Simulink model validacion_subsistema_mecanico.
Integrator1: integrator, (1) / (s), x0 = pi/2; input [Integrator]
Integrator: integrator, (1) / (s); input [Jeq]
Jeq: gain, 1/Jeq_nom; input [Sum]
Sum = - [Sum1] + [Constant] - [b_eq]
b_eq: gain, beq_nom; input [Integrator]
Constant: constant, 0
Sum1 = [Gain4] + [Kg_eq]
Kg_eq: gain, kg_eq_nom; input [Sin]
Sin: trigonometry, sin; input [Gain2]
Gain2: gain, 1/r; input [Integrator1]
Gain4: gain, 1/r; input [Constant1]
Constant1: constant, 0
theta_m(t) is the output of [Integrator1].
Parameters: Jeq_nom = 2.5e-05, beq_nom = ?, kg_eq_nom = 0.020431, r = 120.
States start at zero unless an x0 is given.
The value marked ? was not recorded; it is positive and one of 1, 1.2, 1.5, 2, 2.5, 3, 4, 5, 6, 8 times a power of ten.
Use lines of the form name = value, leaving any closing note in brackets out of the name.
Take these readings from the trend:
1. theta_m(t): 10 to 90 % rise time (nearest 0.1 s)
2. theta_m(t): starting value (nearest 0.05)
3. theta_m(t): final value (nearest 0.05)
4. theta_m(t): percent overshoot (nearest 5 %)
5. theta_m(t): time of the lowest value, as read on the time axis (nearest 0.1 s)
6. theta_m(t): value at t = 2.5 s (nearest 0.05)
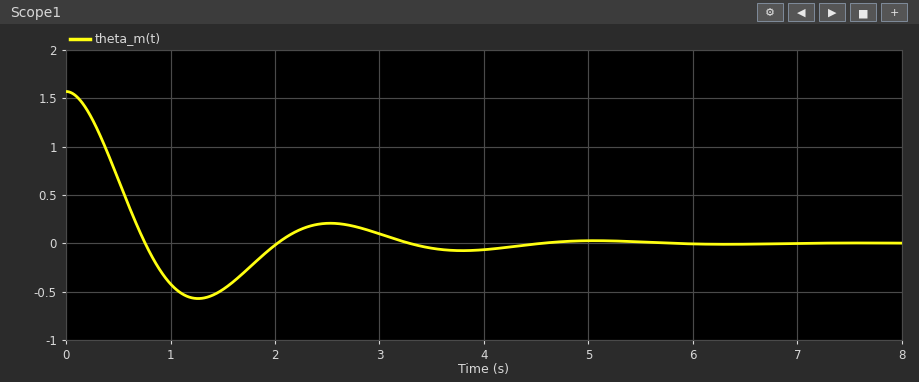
theta_m(t): 10 to 90 % rise time = 0.5 s
theta_m(t): starting value = 1.55
theta_m(t): final value = 0.00
theta_m(t): percent overshoot = 35 %
theta_m(t): time of the lowest value, as read on the time axis = 1.3 s
theta_m(t): value at t = 2.5 s = 0.20
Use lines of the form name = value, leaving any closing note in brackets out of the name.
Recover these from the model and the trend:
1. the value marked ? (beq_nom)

the value marked ? = 4e-05
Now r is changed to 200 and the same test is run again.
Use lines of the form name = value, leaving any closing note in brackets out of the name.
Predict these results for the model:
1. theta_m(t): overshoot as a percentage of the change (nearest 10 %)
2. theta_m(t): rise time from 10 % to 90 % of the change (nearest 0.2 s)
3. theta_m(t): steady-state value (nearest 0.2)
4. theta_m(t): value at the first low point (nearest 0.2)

theta_m(t): overshoot as a percentage of the change = 30 %
theta_m(t): rise time from 10 % to 90 % of the change = 0.8 s
theta_m(t): steady-state value = 0.0
theta_m(t): value at the first low point = -0.4
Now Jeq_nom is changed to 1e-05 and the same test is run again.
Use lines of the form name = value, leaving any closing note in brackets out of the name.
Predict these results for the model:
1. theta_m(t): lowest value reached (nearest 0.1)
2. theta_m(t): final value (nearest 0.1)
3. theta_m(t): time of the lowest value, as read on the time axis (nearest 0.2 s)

theta_m(t): lowest value reached = -0.3
theta_m(t): final value = 0.0
theta_m(t): time of the lowest value, as read on the time axis = 0.8 s
